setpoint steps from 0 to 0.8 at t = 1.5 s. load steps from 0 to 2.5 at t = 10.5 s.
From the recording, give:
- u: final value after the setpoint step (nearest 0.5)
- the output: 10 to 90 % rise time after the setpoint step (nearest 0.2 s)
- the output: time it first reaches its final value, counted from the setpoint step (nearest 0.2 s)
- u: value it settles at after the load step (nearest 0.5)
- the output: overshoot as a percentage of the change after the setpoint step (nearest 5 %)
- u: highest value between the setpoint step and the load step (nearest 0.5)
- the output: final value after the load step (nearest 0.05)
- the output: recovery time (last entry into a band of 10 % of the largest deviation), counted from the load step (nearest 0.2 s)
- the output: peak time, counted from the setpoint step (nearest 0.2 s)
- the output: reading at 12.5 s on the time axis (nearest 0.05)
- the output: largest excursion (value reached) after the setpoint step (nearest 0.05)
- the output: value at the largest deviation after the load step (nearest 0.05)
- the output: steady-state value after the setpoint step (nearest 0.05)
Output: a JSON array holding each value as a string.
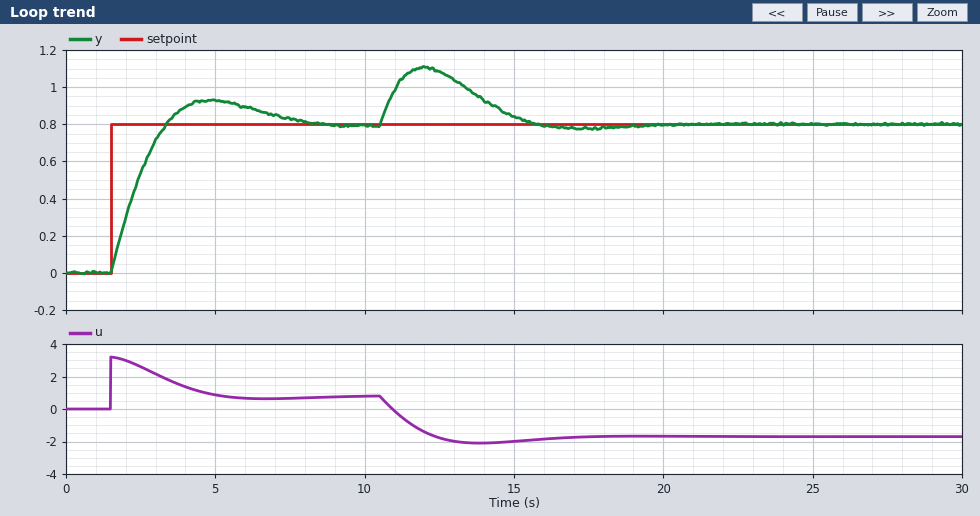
["1.0", "1.4 s", "1.8 s", "-1.5", "15 %", "3.0", "0.80", "4.6 s", "3.4 s", "1.10", "0.95", "1.10", "0.80"]
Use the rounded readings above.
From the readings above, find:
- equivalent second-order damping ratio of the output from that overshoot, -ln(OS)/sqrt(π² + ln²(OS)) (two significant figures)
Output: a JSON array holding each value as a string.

["0.52"]
